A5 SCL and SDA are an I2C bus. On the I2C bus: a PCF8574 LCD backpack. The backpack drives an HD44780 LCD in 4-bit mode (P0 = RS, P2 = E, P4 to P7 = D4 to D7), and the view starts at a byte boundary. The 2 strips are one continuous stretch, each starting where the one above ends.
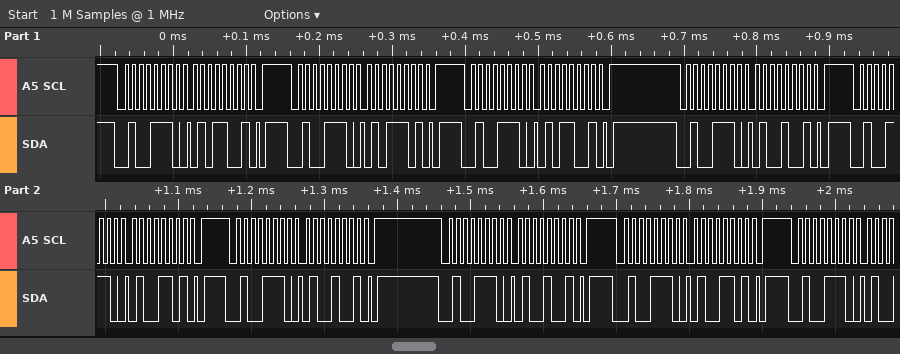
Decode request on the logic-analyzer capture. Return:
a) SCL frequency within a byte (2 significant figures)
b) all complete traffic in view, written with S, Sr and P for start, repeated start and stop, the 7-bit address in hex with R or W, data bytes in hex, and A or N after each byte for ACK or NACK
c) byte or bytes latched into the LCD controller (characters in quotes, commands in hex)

100 kHz
S 27W A 59 A P S 27W A 5D A P S 27W A 59 A P S 27W A 49 A P S 27W A 4D A P S 27W A 49 A P S 27W A 49 A P S 27W A 4D A P S 27W A
'T'
